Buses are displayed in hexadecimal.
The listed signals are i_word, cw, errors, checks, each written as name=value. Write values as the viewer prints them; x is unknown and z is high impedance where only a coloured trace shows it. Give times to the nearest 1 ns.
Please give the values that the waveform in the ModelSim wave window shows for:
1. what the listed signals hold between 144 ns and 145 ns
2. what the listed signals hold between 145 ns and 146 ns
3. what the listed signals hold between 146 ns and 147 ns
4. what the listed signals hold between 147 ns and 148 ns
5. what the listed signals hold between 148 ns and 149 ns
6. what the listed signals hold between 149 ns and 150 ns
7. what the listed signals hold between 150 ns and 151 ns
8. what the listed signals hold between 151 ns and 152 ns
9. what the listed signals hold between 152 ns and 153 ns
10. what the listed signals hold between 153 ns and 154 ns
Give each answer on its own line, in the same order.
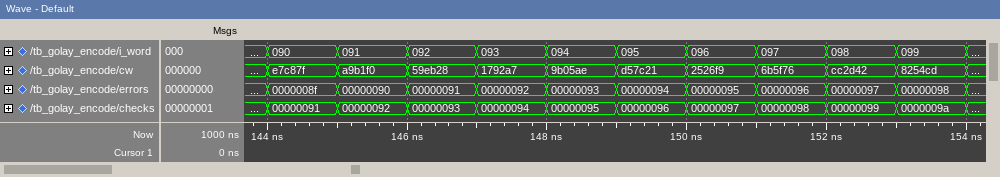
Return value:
i_word=090, cw=e7c87f, errors=0000008f, checks=00000091
i_word=091, cw=a9b1f0, errors=00000090, checks=00000092
i_word=092, cw=59eb28, errors=00000091, checks=00000093
i_word=093, cw=1792a7, errors=00000092, checks=00000094
i_word=094, cw=9b05ae, errors=00000093, checks=00000095
i_word=095, cw=d57c21, errors=00000094, checks=00000096
i_word=096, cw=2526f9, errors=00000095, checks=00000097
i_word=097, cw=6b5f76, errors=00000096, checks=00000098
i_word=098, cw=cc2d42, errors=00000097, checks=00000099
i_word=099, cw=8254cd, errors=00000098, checks=0000009a
